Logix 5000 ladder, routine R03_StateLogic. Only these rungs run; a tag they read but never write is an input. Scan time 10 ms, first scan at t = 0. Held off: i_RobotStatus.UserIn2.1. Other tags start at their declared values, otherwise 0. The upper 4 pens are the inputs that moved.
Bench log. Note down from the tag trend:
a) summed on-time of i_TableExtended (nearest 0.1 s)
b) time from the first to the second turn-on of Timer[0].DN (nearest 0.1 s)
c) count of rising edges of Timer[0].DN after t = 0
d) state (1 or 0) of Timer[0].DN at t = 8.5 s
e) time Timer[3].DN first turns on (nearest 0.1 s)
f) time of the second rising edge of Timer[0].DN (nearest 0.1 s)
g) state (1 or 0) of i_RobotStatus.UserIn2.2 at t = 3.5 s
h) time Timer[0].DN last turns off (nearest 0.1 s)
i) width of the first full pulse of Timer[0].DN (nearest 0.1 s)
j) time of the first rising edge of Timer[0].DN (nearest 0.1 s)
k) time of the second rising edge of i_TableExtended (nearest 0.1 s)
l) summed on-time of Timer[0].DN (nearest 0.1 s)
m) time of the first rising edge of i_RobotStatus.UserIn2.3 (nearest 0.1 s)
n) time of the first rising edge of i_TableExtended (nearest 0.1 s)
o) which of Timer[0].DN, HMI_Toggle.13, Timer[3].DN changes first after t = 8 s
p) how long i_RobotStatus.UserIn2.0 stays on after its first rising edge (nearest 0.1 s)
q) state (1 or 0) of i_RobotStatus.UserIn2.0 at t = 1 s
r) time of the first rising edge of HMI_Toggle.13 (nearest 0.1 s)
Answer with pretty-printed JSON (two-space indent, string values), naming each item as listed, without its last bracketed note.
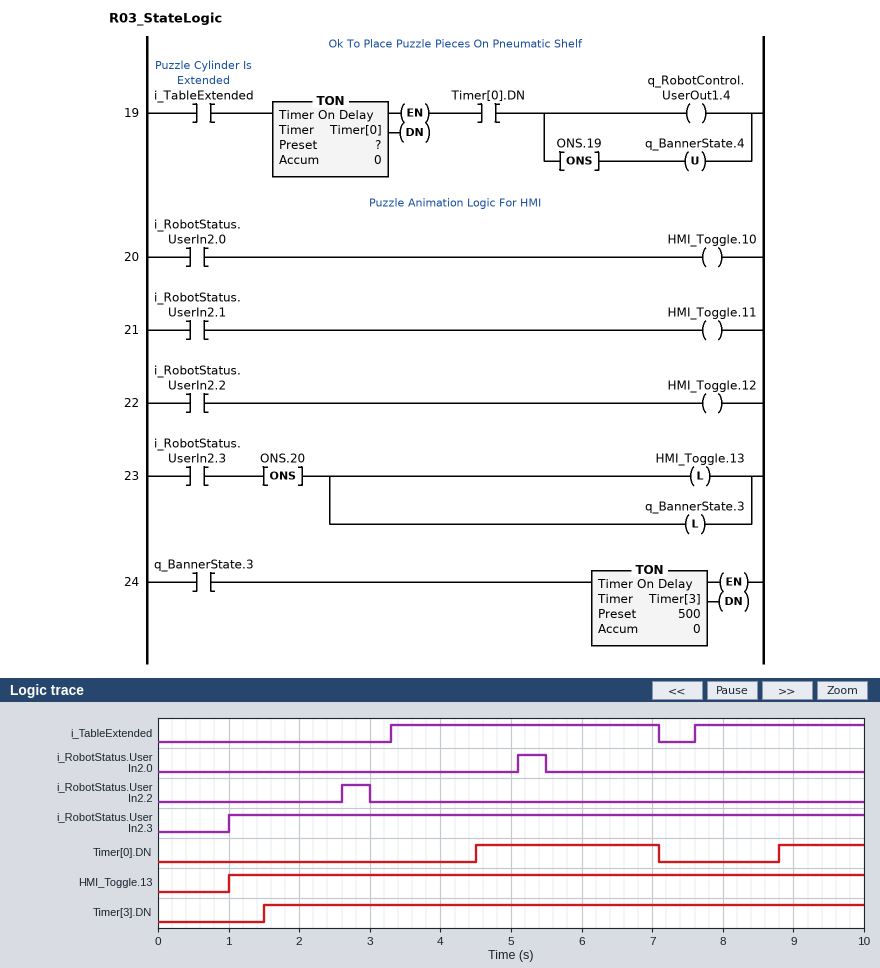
{
  "summed on-time of i_TableExtended": "6.2 s",
  "time from the first to the second turn-on of Timer[0].DN": "4.3 s",
  "count of rising edges of Timer[0].DN after t = 0": "2",
  "state (1 or 0) of Timer[0].DN at t = 8.5 s": "0",
  "time Timer[3].DN first turns on": "1.5 s",
  "time of the second rising edge of Timer[0].DN": "8.8 s",
  "state (1 or 0) of i_RobotStatus.UserIn2.2 at t = 3.5 s": "0",
  "time Timer[0].DN last turns off": "7.1 s",
  "width of the first full pulse of Timer[0].DN": "2.6 s",
  "time of the first rising edge of Timer[0].DN": "4.5 s",
  "time of the second rising edge of i_TableExtended": "7.6 s",
  "summed on-time of Timer[0].DN": "3.8 s",
  "time of the first rising edge of i_RobotStatus.UserIn2.3": "1.0 s",
  "time of the first rising edge of i_TableExtended": "3.3 s",
  "which of Timer[0].DN, HMI_Toggle.13, Timer[3].DN changes first after t = 8 s": "Timer[0].DN",
  "how long i_RobotStatus.UserIn2.0 stays on after its first rising edge": "0.4 s",
  "state (1 or 0) of i_RobotStatus.UserIn2.0 at t = 1 s": "0",
  "time of the first rising edge of HMI_Toggle.13": "1.0 s"
}
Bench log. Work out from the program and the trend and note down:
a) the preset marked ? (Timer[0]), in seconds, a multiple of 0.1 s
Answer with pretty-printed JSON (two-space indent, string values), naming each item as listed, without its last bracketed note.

{
  "the preset marked ? (Timer[0]), in seconds, a multiple of 0.1 s": "1.2 s"
}
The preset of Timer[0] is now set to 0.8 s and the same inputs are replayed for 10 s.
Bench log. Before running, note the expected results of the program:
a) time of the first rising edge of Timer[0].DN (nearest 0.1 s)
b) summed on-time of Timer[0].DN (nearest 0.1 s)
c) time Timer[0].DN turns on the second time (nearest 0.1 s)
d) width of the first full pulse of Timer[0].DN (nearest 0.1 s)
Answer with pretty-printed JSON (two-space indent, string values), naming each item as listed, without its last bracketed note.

{
  "time of the first rising edge of Timer[0].DN": "4.1 s",
  "summed on-time of Timer[0].DN": "4.6 s",
  "time Timer[0].DN turns on the second time": "8.4 s",
  "width of the first full pulse of Timer[0].DN": "3.0 s"
}
